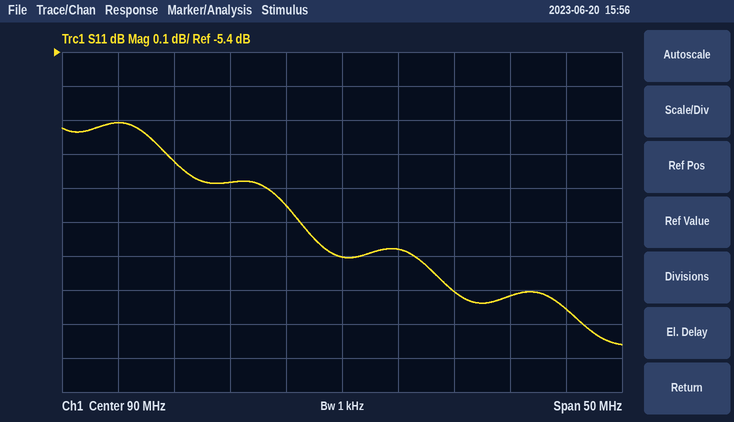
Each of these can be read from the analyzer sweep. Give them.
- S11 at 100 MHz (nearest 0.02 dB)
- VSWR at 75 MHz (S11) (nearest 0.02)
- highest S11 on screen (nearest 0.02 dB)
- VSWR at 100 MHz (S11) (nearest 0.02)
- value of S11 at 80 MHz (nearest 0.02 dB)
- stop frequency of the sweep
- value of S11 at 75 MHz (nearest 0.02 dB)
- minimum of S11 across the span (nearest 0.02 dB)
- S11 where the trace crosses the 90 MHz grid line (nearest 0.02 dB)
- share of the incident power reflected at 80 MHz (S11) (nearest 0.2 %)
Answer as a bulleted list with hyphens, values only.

- -6.10 dB
- 3.14
- -5.60 dB
- 2.96
- -5.78 dB
- 115 MHz
- -5.72 dB
- -6.26 dB
- -6.00 dB
- 26.4 %
